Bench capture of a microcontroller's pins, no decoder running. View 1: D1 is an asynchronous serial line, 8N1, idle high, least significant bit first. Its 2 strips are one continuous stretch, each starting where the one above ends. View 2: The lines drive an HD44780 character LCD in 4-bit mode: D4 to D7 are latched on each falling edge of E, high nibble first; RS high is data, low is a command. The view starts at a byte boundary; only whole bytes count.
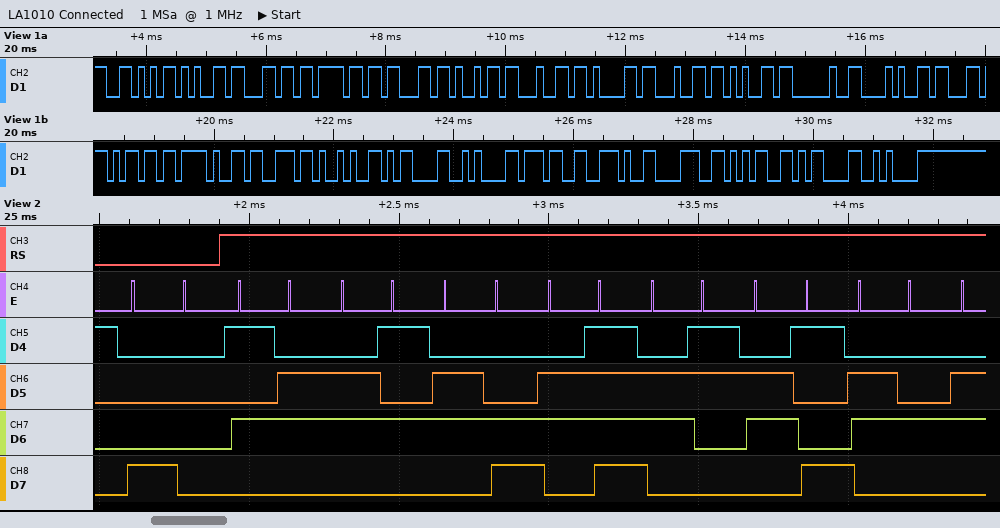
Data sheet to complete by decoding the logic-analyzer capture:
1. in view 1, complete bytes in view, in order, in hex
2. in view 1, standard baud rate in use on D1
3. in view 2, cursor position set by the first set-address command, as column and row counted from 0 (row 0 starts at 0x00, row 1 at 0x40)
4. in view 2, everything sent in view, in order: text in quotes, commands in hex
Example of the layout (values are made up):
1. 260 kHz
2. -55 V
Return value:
1. 56 65 6C 6F 63 69 64 61 64 65 20 28 63 6D 2F 73 29 0D 0A 37 2E 38 35 0D 0A
2. 9600 baud
3. column 0, row 0
4. 0x80 "Velocid"
